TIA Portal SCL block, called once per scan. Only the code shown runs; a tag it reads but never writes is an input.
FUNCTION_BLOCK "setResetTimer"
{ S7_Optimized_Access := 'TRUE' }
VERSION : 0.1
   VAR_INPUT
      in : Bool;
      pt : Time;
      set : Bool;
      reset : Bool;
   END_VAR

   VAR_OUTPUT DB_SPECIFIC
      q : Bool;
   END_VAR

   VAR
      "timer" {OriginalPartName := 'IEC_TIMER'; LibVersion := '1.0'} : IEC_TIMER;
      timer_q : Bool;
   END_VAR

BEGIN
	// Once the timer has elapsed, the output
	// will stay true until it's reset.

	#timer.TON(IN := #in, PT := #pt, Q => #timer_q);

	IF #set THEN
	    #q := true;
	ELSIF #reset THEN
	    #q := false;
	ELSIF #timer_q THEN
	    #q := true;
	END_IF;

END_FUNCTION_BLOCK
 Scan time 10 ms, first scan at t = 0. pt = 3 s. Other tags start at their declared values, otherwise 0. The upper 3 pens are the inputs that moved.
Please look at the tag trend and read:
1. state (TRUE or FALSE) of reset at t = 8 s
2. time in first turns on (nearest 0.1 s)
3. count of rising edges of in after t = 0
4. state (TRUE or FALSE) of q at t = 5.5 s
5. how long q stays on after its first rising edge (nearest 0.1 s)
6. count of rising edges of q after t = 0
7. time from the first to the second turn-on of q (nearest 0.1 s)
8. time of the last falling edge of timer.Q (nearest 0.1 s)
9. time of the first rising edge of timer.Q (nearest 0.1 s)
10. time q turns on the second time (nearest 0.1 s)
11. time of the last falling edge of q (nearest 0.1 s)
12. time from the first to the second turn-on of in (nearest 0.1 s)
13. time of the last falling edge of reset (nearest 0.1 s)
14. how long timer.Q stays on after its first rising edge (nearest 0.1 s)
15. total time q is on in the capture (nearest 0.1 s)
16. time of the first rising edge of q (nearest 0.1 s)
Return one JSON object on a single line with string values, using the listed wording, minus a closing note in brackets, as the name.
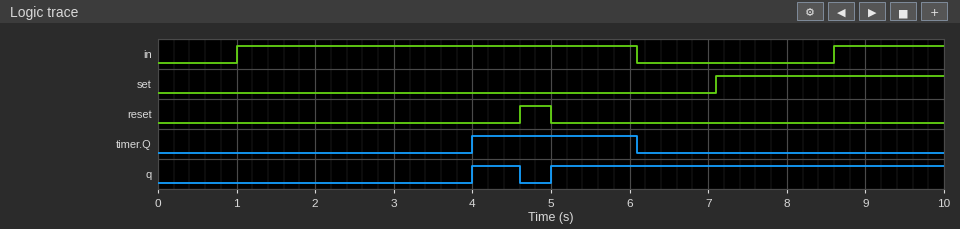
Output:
{"state (TRUE or FALSE) of reset at t = 8 s": "FALSE", "time in first turns on": "1.0 s", "count of rising edges of in after t = 0": "2", "state (TRUE or FALSE) of q at t = 5.5 s": "TRUE", "how long q stays on after its first rising edge": "0.6 s", "count of rising edges of q after t = 0": "2", "time from the first to the second turn-on of q": "1.0 s", "time of the last falling edge of timer.Q": "6.1 s", "time of the first rising edge of timer.Q": "4.0 s", "time q turns on the second time": "5.0 s", "time of the last falling edge of q": "4.6 s", "time from the first to the second turn-on of in": "7.6 s", "time of the last falling edge of reset": "5.0 s", "how long timer.Q stays on after its first rising edge": "2.1 s", "total time q is on in the capture": "5.6 s", "time of the first rising edge of q": "4.0 s"}
